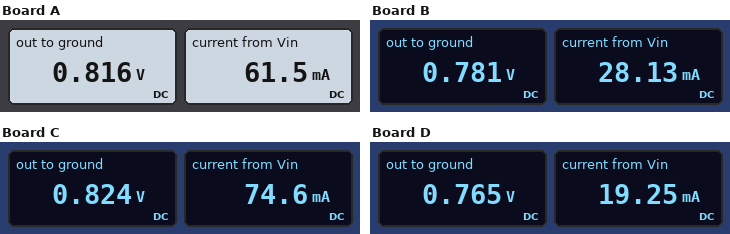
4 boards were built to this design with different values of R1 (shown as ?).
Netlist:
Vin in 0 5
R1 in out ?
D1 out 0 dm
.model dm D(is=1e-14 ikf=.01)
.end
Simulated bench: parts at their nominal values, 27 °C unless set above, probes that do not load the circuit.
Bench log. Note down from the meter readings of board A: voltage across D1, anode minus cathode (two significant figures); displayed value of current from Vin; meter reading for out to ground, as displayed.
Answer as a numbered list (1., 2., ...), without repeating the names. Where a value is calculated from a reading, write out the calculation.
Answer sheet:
1. 816 mV = 820 mV
2. 61.5 mA
3. 0.816 V
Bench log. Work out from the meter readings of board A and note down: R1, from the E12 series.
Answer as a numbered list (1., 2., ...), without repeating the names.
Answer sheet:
1. 68 Ω
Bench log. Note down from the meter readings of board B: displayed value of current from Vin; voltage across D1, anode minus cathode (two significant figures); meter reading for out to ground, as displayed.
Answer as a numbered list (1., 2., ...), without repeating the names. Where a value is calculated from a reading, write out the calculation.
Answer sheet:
1. 28.13 mA
2. 781 mV = 780 mV
3. 0.781 V
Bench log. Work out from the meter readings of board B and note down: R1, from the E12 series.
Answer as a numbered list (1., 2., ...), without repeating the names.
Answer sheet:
1. 150 Ω
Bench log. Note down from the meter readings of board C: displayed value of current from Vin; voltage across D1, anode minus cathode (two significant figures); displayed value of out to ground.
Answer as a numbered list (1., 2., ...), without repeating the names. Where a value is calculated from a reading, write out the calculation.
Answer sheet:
1. 74.6 mA
2. 824 mV = 820 mV
3. 0.824 V
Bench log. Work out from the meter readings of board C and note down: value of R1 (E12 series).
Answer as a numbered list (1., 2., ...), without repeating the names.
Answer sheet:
1. 56 Ω
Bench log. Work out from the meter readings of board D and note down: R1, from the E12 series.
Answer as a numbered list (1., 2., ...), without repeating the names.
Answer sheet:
1. 220 Ω
